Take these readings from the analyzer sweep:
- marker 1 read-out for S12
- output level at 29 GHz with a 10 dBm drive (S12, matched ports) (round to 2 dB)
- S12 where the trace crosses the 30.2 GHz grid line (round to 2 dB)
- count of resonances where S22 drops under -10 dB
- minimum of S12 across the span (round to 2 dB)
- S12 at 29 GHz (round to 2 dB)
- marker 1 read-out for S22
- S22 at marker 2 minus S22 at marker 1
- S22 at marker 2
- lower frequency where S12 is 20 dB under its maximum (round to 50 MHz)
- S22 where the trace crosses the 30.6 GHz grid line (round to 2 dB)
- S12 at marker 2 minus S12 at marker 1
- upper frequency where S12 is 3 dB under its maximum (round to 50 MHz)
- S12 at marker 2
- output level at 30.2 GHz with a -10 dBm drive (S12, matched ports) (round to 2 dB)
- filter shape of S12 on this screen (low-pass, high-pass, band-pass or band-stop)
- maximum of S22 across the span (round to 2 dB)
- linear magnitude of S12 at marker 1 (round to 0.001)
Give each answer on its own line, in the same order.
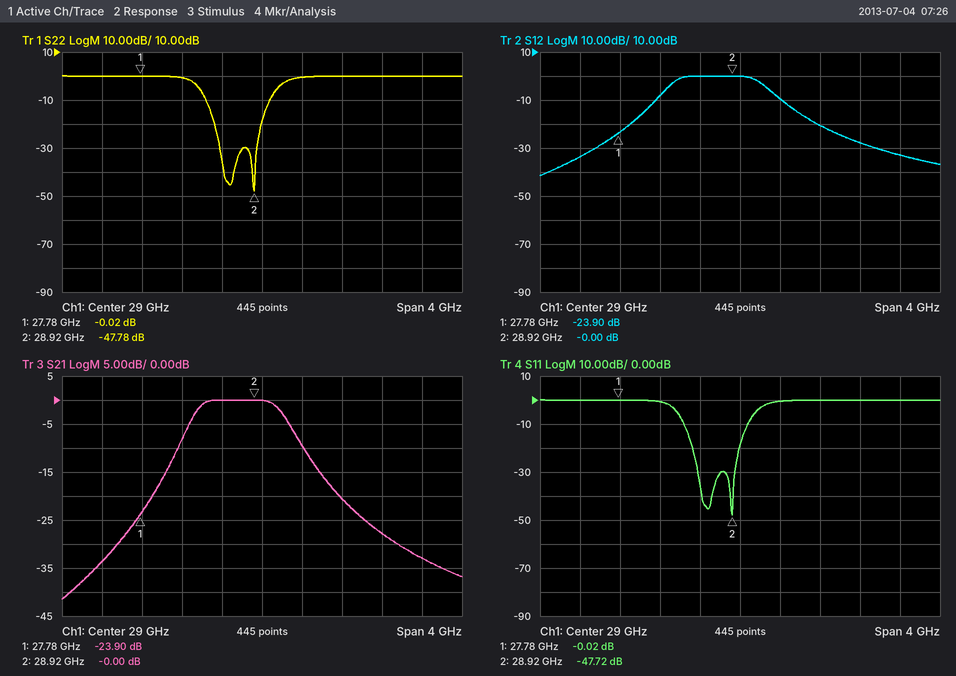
-23.90 dB
10 dBm
-28 dB
2
-42 dB
0 dB
-0.02 dB
-47.76 dB
-47.78 dB
27.90 GHz
0 dB
23.90 dB
29.20 GHz
-0.00 dB
-38 dBm
band-pass
0 dB
0.064
